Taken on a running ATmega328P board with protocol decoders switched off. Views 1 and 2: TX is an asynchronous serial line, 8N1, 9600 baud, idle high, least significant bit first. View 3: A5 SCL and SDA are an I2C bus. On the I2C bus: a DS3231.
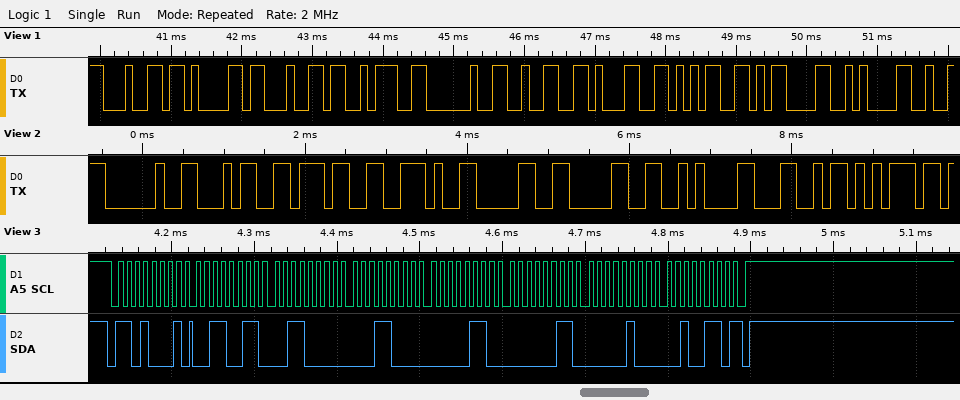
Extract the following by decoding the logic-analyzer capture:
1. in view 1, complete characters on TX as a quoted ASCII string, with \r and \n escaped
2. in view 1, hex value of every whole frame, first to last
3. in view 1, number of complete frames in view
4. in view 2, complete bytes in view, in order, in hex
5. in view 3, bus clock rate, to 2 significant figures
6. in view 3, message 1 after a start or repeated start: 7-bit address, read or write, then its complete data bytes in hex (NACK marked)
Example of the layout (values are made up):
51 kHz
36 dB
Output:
"dad: 215\r\n"
64 61 64 3A 20 32 31 35 0D 0A
10
20 34 37 2E 30 30 0A 4C 75
100 kHz
0x68 read: 33 30 18 06 03 04 26 NACK
